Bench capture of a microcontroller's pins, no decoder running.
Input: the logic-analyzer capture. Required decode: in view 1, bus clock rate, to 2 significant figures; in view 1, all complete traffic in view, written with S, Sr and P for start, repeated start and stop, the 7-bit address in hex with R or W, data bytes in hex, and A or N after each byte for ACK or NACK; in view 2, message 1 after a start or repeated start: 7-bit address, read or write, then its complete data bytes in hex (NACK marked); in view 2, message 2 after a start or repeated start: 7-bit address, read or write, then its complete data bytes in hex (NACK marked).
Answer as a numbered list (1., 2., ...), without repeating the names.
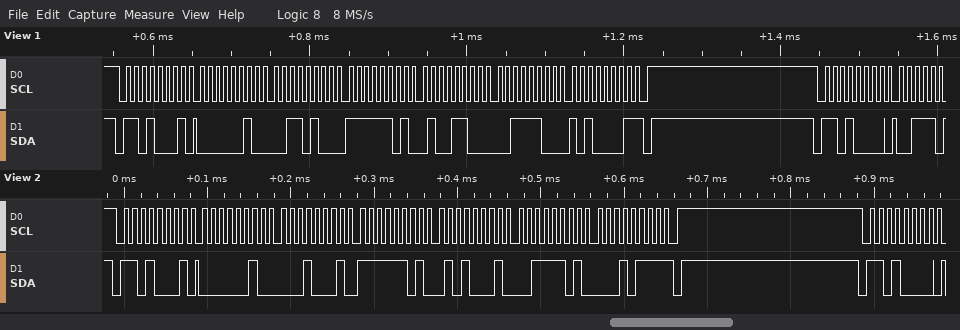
1. 100 kHz
2. S 68R A 02 A 34 A FD A 4C A 3C A A1 N P S 68W A
3. 0x68 read: 02 11 FD 51 3D 17 NACK
4. 0x68 write
